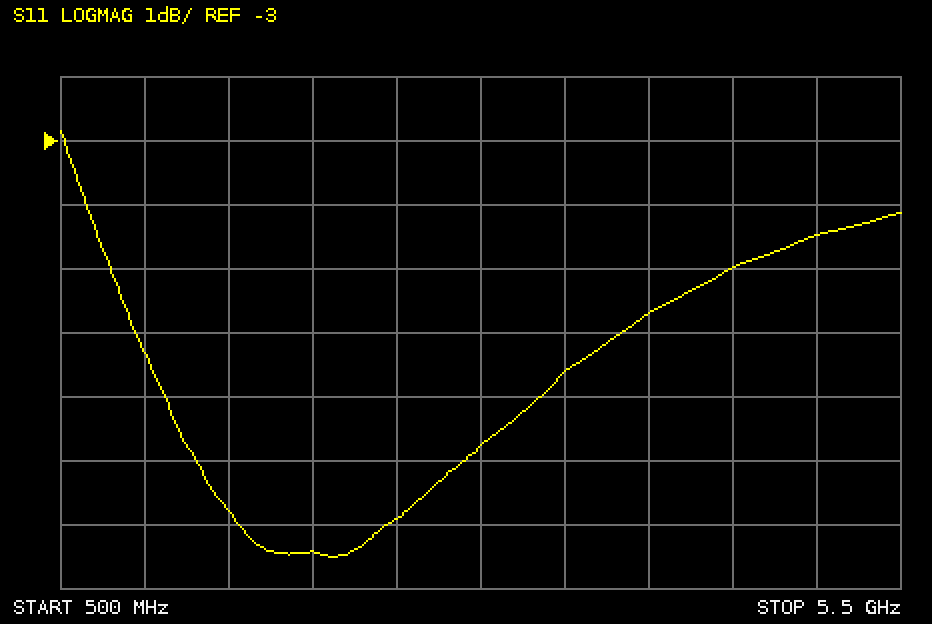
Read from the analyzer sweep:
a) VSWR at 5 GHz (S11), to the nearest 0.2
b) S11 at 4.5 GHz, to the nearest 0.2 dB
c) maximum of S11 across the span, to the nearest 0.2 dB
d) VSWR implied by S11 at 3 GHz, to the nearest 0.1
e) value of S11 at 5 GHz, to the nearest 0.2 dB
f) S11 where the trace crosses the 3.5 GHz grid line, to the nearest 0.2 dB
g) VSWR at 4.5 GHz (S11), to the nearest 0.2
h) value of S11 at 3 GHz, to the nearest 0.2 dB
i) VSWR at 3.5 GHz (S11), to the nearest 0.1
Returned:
4.0
-5.0 dB
-2.8 dB
2.4
-4.4 dB
-6.6 dB
3.6
-7.8 dB
2.8
